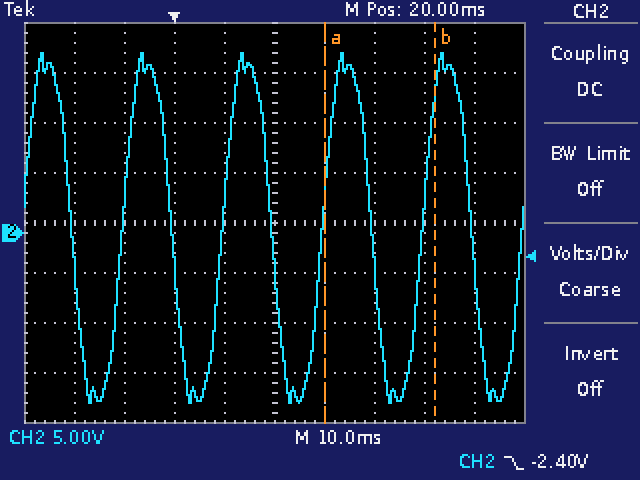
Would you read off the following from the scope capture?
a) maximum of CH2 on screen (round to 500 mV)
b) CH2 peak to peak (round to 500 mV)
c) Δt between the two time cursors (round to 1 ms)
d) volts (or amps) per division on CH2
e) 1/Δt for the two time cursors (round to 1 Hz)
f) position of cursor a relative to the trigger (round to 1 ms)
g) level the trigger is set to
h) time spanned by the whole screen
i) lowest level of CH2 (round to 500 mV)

18.0 V
35.0 V
22 ms
5 V
45 Hz
+30 ms
-2.40 V
100 ms
-17.0 V
